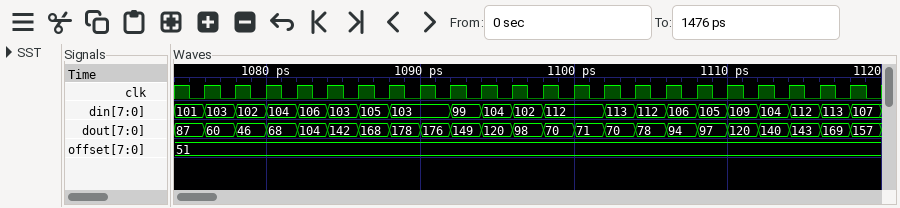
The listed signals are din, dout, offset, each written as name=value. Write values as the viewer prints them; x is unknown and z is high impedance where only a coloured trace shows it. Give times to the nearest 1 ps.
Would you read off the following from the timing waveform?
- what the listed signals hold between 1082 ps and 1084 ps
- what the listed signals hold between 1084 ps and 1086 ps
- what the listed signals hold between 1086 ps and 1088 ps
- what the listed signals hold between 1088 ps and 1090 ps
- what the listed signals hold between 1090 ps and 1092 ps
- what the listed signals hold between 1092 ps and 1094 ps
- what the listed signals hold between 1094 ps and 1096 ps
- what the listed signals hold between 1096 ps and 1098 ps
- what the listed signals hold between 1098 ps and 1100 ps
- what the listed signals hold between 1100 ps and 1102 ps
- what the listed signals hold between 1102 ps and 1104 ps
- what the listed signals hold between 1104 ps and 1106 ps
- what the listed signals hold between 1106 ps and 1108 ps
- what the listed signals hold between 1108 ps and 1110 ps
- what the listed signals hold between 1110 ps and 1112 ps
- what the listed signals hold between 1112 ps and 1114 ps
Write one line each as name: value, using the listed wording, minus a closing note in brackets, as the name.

what the listed signals hold between 1082 ps and 1084 ps: din=106, dout=104, offset=51
what the listed signals hold between 1084 ps and 1086 ps: din=103, dout=142, offset=51
what the listed signals hold between 1086 ps and 1088 ps: din=105, dout=168, offset=51
what the listed signals hold between 1088 ps and 1090 ps: din=103, dout=178, offset=51
what the listed signals hold between 1090 ps and 1092 ps: din=103, dout=176, offset=51
what the listed signals hold between 1092 ps and 1094 ps: din=99, dout=149, offset=51
what the listed signals hold between 1094 ps and 1096 ps: din=104, dout=120, offset=51
what the listed signals hold between 1096 ps and 1098 ps: din=102, dout=98, offset=51
what the listed signals hold between 1098 ps and 1100 ps: din=112, dout=70, offset=51
what the listed signals hold between 1100 ps and 1102 ps: din=112, dout=71, offset=51
what the listed signals hold between 1102 ps and 1104 ps: din=113, dout=70, offset=51
what the listed signals hold between 1104 ps and 1106 ps: din=112, dout=78, offset=51
what the listed signals hold between 1106 ps and 1108 ps: din=106, dout=94, offset=51
what the listed signals hold between 1108 ps and 1110 ps: din=105, dout=97, offset=51
what the listed signals hold between 1110 ps and 1112 ps: din=109, dout=120, offset=51
what the listed signals hold between 1112 ps and 1114 ps: din=104, dout=140, offset=51
